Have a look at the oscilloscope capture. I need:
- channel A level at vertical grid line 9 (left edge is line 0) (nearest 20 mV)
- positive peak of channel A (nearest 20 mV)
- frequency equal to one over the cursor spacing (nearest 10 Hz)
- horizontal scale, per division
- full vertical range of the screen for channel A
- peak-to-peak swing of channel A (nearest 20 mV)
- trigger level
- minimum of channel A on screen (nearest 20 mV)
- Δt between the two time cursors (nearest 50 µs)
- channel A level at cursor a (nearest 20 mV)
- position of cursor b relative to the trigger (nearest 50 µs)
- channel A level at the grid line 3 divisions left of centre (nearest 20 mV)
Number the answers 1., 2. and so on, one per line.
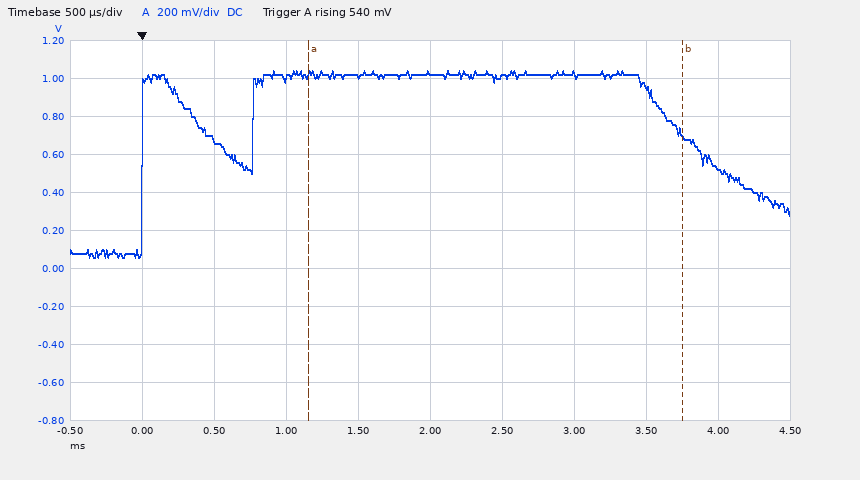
1. 520 mV
2. 1.04 V
3. 380 Hz
4. 500 µs
5. 2 V
6. 980 mV
7. 540 mV
8. 60 mV
9. 2.60 ms
10. 1.02 V
11. +3.75 ms
12. 680 mV
